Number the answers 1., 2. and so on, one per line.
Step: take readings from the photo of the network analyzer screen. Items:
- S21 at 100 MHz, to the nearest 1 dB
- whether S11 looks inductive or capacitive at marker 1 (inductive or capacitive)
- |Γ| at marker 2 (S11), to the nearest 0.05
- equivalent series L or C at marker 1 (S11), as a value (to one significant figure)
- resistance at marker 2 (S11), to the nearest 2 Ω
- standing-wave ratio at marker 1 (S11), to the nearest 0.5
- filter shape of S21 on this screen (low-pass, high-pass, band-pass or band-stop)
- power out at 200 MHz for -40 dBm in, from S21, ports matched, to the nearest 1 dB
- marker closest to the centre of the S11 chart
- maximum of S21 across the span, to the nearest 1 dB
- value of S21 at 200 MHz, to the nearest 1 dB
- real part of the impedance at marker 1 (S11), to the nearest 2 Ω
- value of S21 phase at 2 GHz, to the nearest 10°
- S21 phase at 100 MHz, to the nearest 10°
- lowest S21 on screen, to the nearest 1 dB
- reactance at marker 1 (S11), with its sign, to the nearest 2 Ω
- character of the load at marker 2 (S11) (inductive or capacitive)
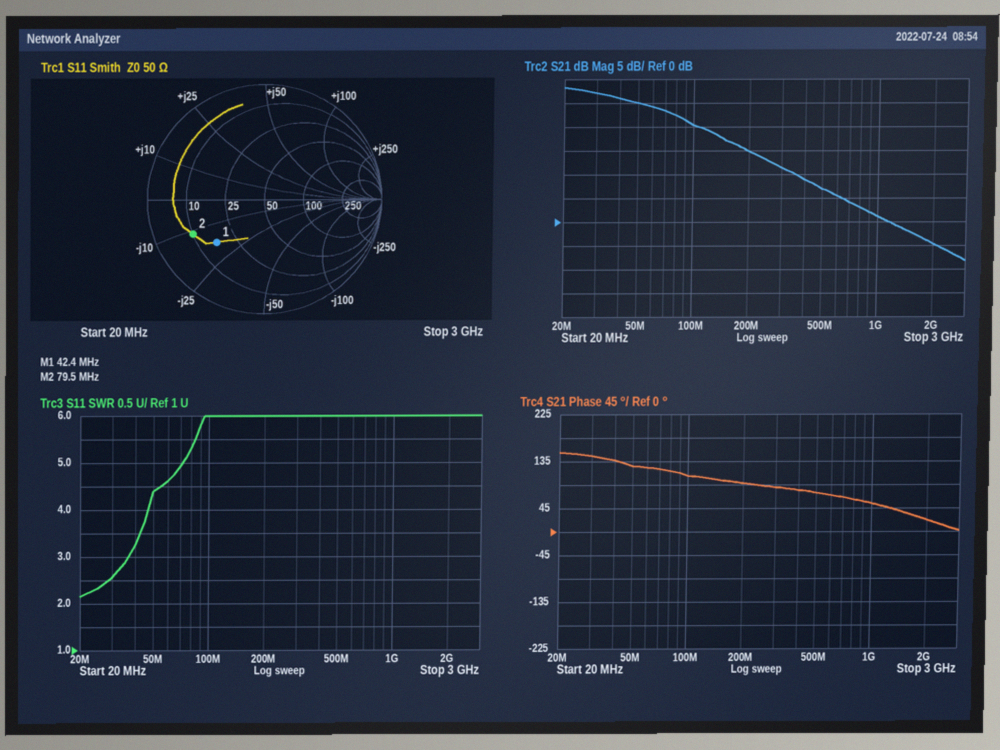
1. 20 dB
2. capacitive
3. 0.70
4. 200 pF
5. 10 Ω
6. 3.5
7. low-pass
8. -25 dBm
9. marker 1
10. 28 dB
11. 15 dB
12. 16 Ω
13. 20°
14. 110°
15. -8 dB
16. -18 Ω
17. capacitive
